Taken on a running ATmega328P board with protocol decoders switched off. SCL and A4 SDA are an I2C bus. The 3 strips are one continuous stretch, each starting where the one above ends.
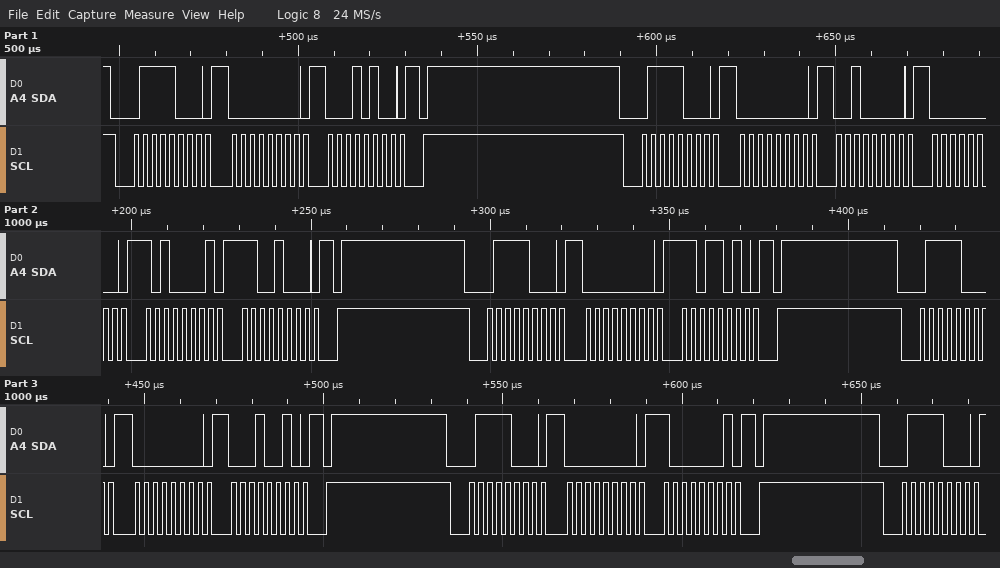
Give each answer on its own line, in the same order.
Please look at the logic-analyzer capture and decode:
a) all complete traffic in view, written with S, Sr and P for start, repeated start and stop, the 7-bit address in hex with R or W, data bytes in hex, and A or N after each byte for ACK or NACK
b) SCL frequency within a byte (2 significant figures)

S 3CW A 00 A 14 A P S 3CW A 00 A 20 A 00 A A1 A C8 A P S 3CW A 00 A DA A P S 3CW A 00 A 12 A P S 3CW A 00 A 81 A P S 3CW A
400 kHz
